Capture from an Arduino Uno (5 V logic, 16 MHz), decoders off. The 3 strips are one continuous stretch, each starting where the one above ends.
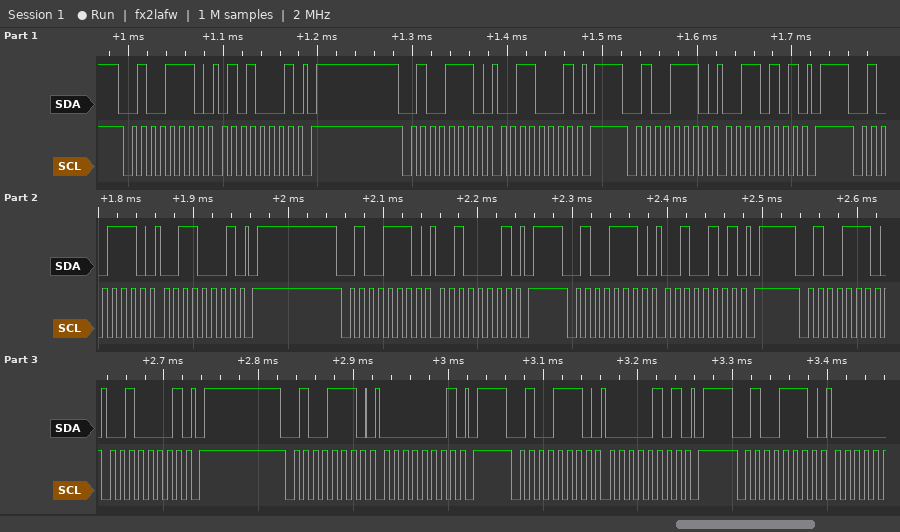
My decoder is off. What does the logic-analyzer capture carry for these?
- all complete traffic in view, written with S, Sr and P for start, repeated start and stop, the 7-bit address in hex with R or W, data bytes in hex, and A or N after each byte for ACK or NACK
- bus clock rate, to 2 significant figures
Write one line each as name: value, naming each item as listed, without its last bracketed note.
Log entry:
all complete traffic in view, written with S, Sr and P for start, repeated start and stop, the 7-bit address in hex with R or W, data bytes in hex, and A or N after each byte for ACK or NACK: S 27W A 51 A P S 27W A 31 A P S 27W A 35 A P S 27W A 31 A P S 27W A 21 A P S 27W A 25 A P S 27W A 21 A P S 27W A 01 A P S 27W A 05 A P S 27W A
bus clock rate, to 2 significant figures: 100 kHz
